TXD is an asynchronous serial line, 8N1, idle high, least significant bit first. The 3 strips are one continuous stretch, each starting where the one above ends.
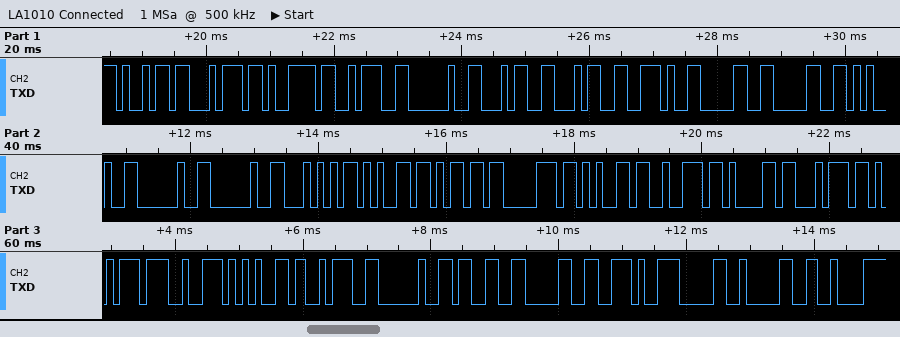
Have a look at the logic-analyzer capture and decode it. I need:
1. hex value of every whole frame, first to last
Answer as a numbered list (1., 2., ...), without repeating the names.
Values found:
1. 69 74 79 3A 20 34 34 2E 30 30 25 20 20 54 65 6D 70 65 72 61 74 75 72 65 3A 20 33 30 2E 30 30 C2
